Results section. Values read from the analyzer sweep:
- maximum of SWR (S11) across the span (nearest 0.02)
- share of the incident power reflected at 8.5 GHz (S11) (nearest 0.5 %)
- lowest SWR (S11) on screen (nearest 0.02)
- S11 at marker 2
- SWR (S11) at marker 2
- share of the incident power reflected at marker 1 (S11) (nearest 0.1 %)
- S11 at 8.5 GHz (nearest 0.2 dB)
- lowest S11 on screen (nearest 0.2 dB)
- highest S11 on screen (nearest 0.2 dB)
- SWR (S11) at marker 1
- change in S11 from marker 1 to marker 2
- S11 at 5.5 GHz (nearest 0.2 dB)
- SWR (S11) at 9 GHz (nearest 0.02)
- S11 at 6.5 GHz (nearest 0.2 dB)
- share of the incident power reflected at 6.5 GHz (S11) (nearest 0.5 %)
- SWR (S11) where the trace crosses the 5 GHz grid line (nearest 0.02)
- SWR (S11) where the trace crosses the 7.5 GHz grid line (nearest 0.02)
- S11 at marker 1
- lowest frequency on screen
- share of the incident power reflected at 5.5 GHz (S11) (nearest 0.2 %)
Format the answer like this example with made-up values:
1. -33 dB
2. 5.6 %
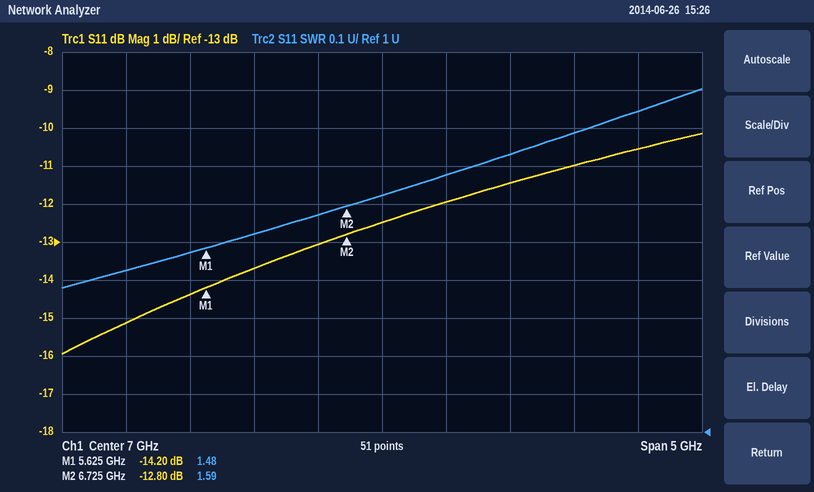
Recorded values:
1. 1.90
2. 8.0 %
3. 1.38
4. -12.80 dB
5. 1.59
6. 3.8 %
7. -11.0 dB
8. -16.0 dB
9. -10.2 dB
10. 1.48
11. 1.40 dB
12. -14.4 dB
13. 1.84
14. -13.0 dB
15. 5.0 %
16. 1.42
17. 1.68
18. -14.20 dB
19. 4.5 GHz
20. 3.6 %
